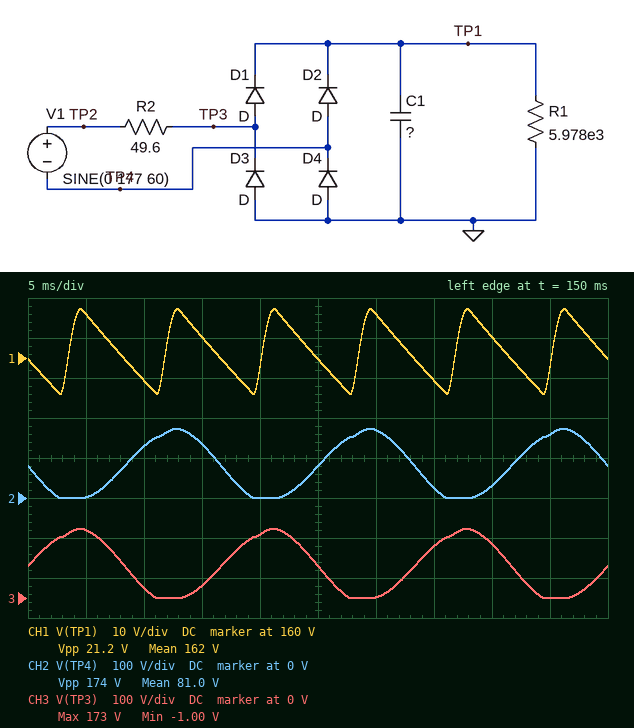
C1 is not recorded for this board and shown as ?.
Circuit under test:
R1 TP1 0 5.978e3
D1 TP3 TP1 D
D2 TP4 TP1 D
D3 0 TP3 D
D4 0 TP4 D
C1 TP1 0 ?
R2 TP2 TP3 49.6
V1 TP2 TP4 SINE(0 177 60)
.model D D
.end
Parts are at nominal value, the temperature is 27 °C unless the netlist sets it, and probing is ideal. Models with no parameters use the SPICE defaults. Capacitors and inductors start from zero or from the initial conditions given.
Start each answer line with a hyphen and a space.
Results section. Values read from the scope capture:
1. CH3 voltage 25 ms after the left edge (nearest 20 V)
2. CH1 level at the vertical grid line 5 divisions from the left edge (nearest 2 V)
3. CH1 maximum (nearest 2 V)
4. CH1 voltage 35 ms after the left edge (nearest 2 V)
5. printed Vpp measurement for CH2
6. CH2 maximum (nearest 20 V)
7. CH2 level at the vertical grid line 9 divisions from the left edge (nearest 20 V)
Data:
- 80 V
- 160 V
- 172 V
- 154 V
- 174 V
- 180 V
- 160 V
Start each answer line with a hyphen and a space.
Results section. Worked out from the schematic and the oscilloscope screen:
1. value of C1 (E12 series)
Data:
- 8.2 µF
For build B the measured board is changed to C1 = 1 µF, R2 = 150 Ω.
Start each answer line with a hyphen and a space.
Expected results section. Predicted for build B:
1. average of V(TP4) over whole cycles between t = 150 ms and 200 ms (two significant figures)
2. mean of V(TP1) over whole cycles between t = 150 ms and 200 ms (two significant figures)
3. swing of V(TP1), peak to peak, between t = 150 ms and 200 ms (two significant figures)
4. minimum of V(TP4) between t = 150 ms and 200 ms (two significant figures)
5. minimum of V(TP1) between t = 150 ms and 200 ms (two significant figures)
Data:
- 64 V
- 130 V
- 93 V
- -760 mV
- 78 V
